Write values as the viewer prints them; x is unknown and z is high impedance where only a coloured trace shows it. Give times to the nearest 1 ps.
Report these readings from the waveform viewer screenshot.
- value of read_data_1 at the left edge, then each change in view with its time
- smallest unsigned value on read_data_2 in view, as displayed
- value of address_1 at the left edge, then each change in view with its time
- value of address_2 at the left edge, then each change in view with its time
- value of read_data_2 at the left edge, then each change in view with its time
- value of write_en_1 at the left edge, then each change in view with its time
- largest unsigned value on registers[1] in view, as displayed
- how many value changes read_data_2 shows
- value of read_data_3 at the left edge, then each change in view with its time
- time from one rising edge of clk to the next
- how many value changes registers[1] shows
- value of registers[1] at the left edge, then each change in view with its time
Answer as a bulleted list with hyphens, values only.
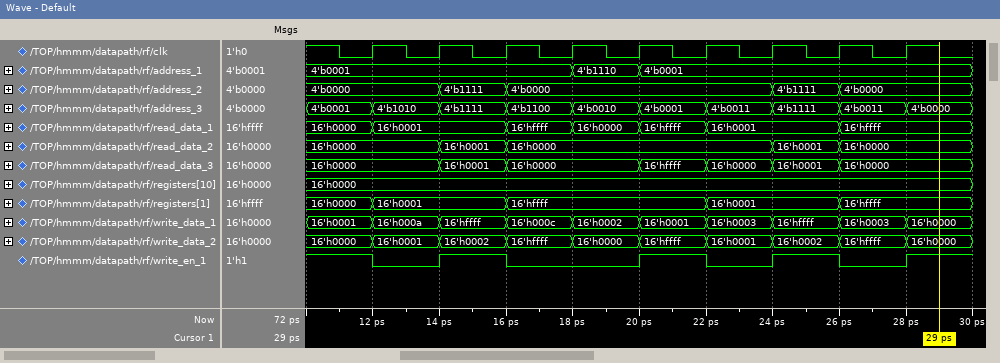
- 16'h0000, 16'h0001 at 12 ps, 16'hffff at 16 ps, 16'h0000 at 18 ps, 16'hffff at 20 ps, 16'h0001 at 22 ps, 16'hffff at 26 ps
- 16'h0000
- 4'b0001, 4'b1110 at 18 ps, 4'b0001 at 20 ps
- 4'b0000, 4'b1111 at 14 ps, 4'b0000 at 16 ps, 4'b1111 at 24 ps, 4'b0000 at 26 ps
- 16'h0000, 16'h0001 at 14 ps, 16'h0000 at 16 ps, 16'h0001 at 24 ps, 16'h0000 at 26 ps
- 1, 0 at 12 ps, 1 at 14 ps, 0 at 16 ps, 1 at 20 ps, 0 at 22 ps, 1 at 24 ps, 0 at 26 ps, 1 at 28 ps
- 16'hffff
- 4
- 16'h0000, 16'h0001 at 14 ps, 16'h0000 at 16 ps, 16'hffff at 20 ps, 16'h0000 at 22 ps, 16'h0001 at 24 ps, 16'h0000 at 26 ps
- 2 ps
- 4
- 16'h0000, 16'h0001 at 12 ps, 16'hffff at 16 ps, 16'h0001 at 22 ps, 16'hffff at 26 ps
